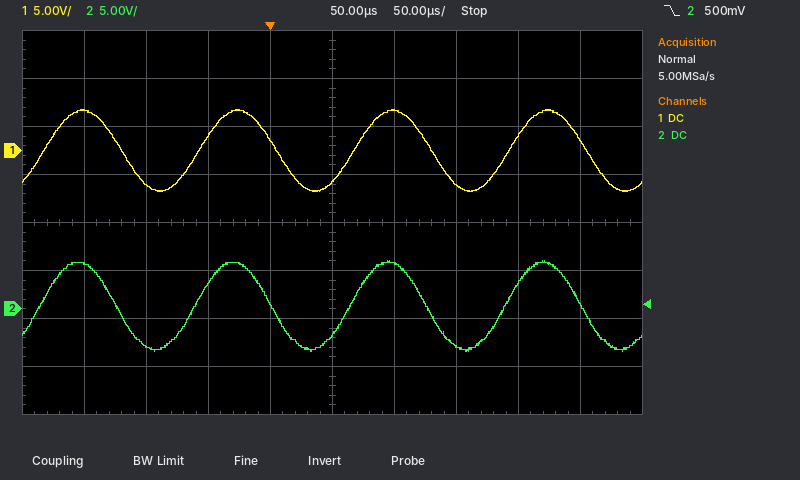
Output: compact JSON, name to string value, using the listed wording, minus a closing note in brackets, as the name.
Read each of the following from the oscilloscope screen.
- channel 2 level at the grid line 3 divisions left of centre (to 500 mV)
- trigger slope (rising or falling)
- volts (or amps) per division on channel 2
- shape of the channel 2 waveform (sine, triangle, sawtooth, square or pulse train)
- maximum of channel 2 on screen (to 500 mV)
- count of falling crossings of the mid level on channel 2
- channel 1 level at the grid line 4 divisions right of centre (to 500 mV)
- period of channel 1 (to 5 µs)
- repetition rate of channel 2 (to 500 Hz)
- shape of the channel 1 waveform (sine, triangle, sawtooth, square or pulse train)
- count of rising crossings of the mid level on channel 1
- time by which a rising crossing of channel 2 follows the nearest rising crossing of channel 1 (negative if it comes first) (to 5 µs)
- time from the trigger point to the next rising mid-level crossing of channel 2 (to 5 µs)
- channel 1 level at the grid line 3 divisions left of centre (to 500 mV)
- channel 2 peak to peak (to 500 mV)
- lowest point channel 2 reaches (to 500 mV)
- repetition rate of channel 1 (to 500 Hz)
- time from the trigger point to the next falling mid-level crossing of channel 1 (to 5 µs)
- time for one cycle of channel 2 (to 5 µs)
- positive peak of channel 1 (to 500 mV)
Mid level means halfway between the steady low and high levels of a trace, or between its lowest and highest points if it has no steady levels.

{"channel 2 level at the grid line 3 divisions left of centre": "-4.0 V", "trigger slope": "falling", "volts (or amps) per division on channel 2": "5 V", "shape of the channel 2 waveform": "sine", "maximum of channel 2 on screen": "5.0 V", "count of falling crossings of the mid level on channel 2": "4", "channel 1 level at the grid line 4 divisions right of centre": "1.0 V", "period of channel 1": "125 µs", "repetition rate of channel 2": "8.0 kHz", "shape of the channel 1 waveform": "sine", "count of rising crossings of the mid level on channel 1": "4", "time by which a rising crossing of channel 2 follows the nearest rising crossing of channel 1 (negative if it comes first)": "-5 µs", "time from the trigger point to the next rising mid-level crossing of channel 2": "65 µs", "channel 1 level at the grid line 3 divisions left of centre": "-3.5 V", "channel 2 peak to peak": "9.5 V", "lowest point channel 2 reaches": "-4.5 V", "repetition rate of channel 1": "8.0 kHz", "time from the trigger point to the next falling mid-level crossing of channel 1": "5 µs", "time for one cycle of channel 2": "125 µs", "positive peak of channel 1": "4.5 V"}
